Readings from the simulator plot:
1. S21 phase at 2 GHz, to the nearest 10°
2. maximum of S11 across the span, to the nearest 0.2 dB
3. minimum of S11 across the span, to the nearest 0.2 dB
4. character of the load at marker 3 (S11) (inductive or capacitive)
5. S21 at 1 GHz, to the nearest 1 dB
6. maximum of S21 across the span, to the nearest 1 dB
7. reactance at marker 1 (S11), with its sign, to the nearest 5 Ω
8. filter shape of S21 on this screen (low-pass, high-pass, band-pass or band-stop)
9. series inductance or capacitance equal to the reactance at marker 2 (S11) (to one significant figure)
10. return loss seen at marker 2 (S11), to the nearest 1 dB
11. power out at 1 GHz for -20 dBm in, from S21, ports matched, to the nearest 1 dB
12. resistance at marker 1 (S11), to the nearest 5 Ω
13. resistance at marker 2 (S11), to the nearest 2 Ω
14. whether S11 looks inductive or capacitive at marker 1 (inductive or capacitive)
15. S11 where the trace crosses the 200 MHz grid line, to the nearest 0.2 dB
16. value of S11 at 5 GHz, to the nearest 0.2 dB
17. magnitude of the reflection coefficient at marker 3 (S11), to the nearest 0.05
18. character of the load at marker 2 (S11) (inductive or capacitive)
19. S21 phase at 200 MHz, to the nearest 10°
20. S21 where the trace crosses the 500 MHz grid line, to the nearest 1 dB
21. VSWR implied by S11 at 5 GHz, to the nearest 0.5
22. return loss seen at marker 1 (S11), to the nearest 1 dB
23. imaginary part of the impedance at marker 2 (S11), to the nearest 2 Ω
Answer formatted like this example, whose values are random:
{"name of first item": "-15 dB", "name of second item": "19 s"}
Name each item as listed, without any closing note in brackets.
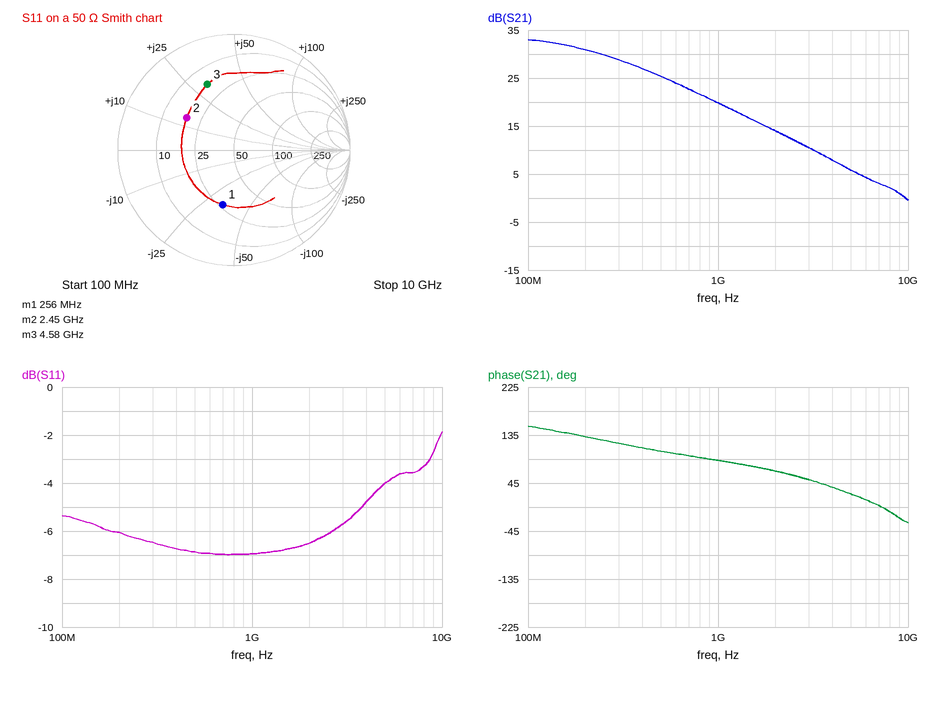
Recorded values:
{"S21 phase at 2 GHz, to the nearest 10°": "70°", "maximum of S11 across the span, to the nearest 0.2 dB": "-1.8 dB", "minimum of S11 across the span, to the nearest 0.2 dB": "-7.0 dB", "character of the load at marker 3 (S11)": "inductive", "S21 at 1 GHz, to the nearest 1 dB": "20 dB", "maximum of S21 across the span, to the nearest 1 dB": "33 dB", "reactance at marker 1 (S11), with its sign, to the nearest 5 Ω": "-35 Ω", "filter shape of S21 on this screen": "low-pass", "series inductance or capacitance equal to the reactance at marker 2 (S11)": "900 pH", "return loss seen at marker 2 (S11), to the nearest 1 dB": "6 dB", "power out at 1 GHz for -20 dBm in, from S21, ports matched, to the nearest 1 dB": "0 dBm", "resistance at marker 1 (S11), to the nearest 5 Ω": "25 Ω", "resistance at marker 2 (S11), to the nearest 2 Ω": "18 Ω", "whether S11 looks inductive or capacitive at marker 1": "capacitive", "S11 where the trace crosses the 200 MHz grid line, to the nearest 0.2 dB": "-6.0 dB", "value of S11 at 5 GHz, to the nearest 0.2 dB": "-4.0 dB", "magnitude of the reflection coefficient at marker 3 (S11), to the nearest 0.05": "0.60", "character of the load at marker 2 (S11)": "inductive", "S21 phase at 200 MHz, to the nearest 10°": "130°", "S21 where the trace crosses the 500 MHz grid line, to the nearest 1 dB": "25 dB", "VSWR implied by S11 at 5 GHz, to the nearest 0.5": "4.5", "return loss seen at marker 1 (S11), to the nearest 1 dB": "6 dB", "imaginary part of the impedance at marker 2 (S11), to the nearest 2 Ω": "+14 Ω"}
